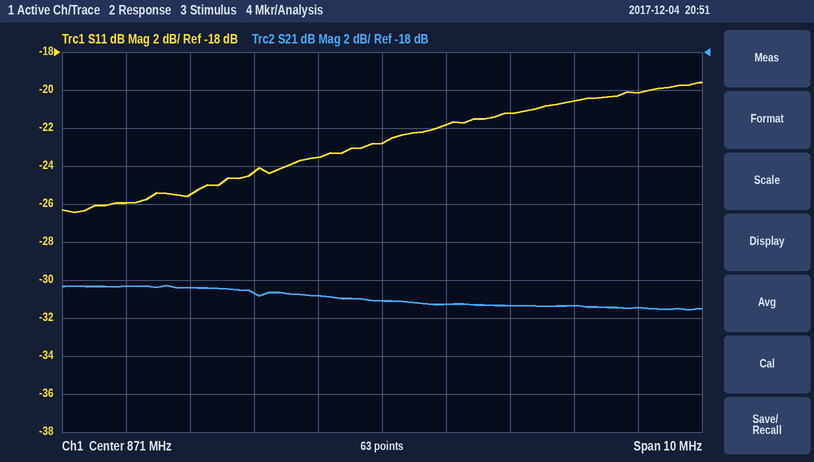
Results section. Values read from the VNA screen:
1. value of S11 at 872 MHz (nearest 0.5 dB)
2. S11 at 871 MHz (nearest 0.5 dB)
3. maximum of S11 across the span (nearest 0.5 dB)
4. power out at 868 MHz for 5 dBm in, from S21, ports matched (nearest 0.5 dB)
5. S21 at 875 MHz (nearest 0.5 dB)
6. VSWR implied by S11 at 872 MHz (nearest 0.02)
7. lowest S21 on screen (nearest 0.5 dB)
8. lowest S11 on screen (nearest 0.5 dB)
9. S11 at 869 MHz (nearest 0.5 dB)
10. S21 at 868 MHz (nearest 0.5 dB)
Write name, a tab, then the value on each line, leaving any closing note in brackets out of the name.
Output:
value of S11 at 872 MHz	-22.0 dB
S11 at 871 MHz	-23.0 dB
maximum of S11 across the span	-19.5 dB
power out at 868 MHz for 5 dBm in, from S21, ports matched	-25.5 dBm
S21 at 875 MHz	-31.5 dB
VSWR implied by S11 at 872 MHz	1.18
lowest S21 on screen	-31.5 dB
lowest S11 on screen	-26.5 dB
S11 at 869 MHz	-24.5 dB
S21 at 868 MHz	-30.5 dB
